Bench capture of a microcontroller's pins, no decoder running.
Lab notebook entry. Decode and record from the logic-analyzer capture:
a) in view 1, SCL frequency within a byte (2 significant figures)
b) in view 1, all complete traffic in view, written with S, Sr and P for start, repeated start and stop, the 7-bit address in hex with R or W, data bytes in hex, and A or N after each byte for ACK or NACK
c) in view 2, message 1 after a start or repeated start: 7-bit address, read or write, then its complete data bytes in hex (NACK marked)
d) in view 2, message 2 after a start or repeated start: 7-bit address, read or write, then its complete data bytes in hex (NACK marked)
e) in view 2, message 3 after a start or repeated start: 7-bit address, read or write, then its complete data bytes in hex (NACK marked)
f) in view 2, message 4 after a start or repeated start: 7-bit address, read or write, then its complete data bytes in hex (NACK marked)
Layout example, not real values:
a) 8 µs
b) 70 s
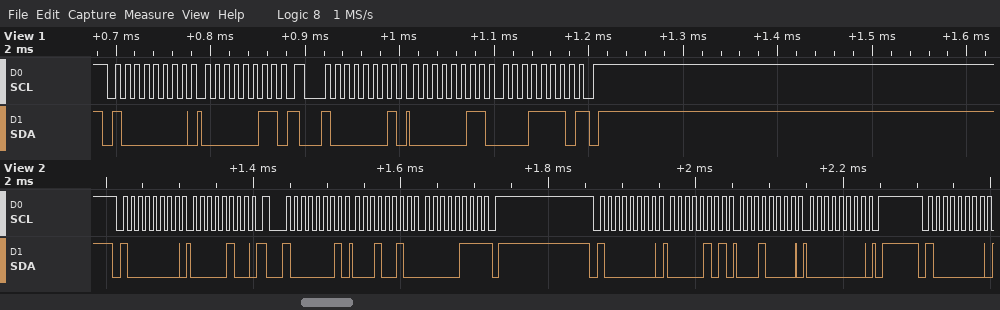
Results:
a) 100 kHz
b) S 40W A 03 A Sr 40R A 03 A 1E N P
c) 0x40 write: 04
d) 0x40 read: 12 07 NACK
e) 0x40 write: 05 10 00
f) 0x40 write
